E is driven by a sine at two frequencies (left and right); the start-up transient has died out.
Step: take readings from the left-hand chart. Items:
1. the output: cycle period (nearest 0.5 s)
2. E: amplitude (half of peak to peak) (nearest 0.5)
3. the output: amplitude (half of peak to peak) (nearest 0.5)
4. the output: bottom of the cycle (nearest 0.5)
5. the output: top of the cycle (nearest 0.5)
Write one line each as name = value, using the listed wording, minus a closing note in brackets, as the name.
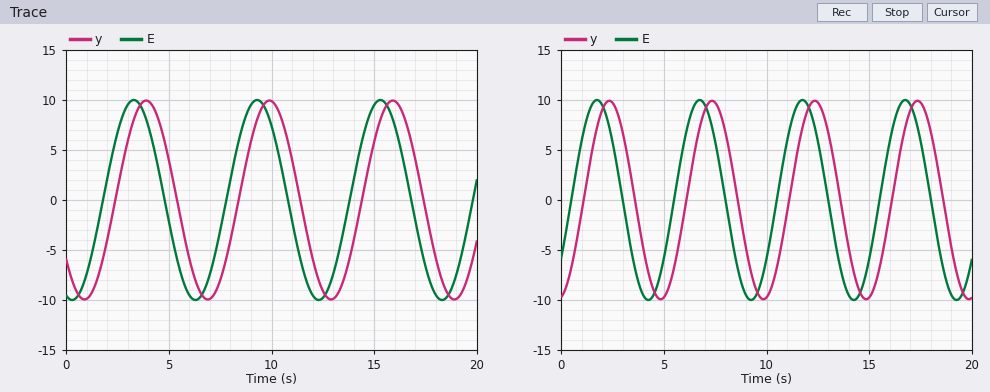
the output: cycle period = 6.0 s
E: amplitude (half of peak to peak) = 10.0
the output: amplitude (half of peak to peak) = 10.0
the output: bottom of the cycle = -10.0
the output: top of the cycle = 10.0
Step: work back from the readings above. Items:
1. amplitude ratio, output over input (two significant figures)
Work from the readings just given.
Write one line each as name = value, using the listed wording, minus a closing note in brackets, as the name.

amplitude ratio, output over input = 1.0
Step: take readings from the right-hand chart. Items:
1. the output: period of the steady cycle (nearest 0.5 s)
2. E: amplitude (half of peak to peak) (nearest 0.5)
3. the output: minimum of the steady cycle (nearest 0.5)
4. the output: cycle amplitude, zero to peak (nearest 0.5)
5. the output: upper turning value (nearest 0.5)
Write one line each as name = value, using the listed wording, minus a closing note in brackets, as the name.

the output: period of the steady cycle = 5.0 s
E: amplitude (half of peak to peak) = 10.0
the output: minimum of the steady cycle = -10.0
the output: cycle amplitude, zero to peak = 10.0
the output: upper turning value = 10.0
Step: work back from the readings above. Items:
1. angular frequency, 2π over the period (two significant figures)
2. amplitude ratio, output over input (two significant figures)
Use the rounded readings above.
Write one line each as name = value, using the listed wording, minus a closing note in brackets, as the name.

angular frequency, 2π over the period = 1.3 rad/s
amplitude ratio, output over input = 1.0
